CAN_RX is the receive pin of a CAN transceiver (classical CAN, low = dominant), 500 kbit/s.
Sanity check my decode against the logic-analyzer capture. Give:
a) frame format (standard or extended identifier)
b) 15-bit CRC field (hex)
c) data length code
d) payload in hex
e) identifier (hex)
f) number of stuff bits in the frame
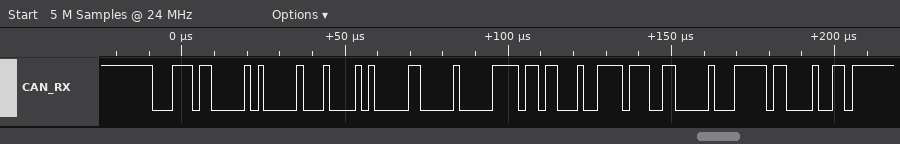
standard
0x7F09
8
04 28 20 07 6C 4F 73 00
0x1D8
7
